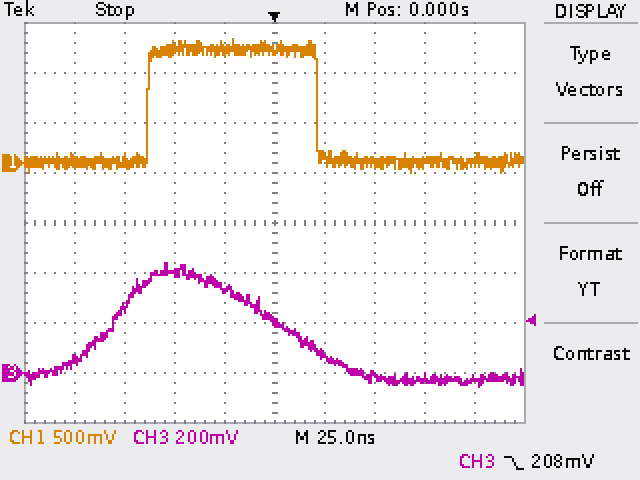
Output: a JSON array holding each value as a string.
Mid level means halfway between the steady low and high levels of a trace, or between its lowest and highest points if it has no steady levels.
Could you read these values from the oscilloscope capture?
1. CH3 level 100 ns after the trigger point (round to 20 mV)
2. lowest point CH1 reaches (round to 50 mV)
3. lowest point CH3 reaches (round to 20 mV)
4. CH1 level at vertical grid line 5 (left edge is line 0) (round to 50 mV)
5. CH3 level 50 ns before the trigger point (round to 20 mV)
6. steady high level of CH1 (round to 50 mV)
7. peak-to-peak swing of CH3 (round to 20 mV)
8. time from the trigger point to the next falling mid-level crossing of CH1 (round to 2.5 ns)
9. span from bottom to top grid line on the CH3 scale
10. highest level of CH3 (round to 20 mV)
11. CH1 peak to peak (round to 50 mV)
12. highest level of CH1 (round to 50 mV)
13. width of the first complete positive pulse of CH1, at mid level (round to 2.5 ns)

["-20 mV", "-100 mV", "-60 mV", "1.15 V", "400 mV", "1.15 V", "500 mV", "22.5 ns", "1.6 V", "440 mV", "1.35 V", "1.25 V", "85.0 ns"]
